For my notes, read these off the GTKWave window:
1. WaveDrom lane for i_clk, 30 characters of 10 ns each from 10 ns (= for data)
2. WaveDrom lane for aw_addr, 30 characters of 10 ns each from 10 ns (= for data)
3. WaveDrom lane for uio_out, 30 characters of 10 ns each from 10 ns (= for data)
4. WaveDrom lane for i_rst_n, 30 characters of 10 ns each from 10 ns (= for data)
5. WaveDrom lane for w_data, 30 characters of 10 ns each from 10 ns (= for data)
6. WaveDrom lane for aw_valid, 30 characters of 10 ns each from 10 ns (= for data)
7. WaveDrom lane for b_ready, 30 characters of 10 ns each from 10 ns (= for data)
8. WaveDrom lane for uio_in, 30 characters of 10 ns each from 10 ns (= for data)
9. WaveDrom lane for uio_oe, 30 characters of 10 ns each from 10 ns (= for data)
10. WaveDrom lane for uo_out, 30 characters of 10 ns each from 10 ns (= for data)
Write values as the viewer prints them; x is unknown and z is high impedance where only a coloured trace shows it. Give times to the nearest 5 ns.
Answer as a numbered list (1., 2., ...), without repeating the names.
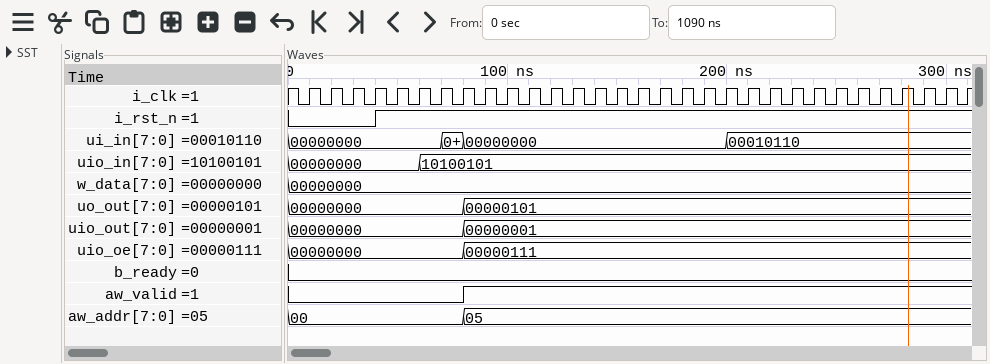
1. {name: 'i_clk', wave: 'p.............................'}
2. {name: 'aw_addr', wave: '=......=......................', data: '00 05'}
3. {name: 'uio_out', wave: '=......=......................', data: '00000000 00000001'}
4. {name: 'i_rst_n', wave: '0..1..........................'}
5. {name: 'w_data', wave: '=.............................', data: '00000000'}
6. {name: 'aw_valid', wave: '0......1......................'}
7. {name: 'b_ready', wave: '0.............................'}
8. {name: 'uio_in', wave: '=....=........................', data: '00000000 10100101'}
9. {name: 'uio_oe', wave: '=......=......................', data: '00000000 00000111'}
10. {name: 'uo_out', wave: '=......=......................', data: '00000000 00000101'}
